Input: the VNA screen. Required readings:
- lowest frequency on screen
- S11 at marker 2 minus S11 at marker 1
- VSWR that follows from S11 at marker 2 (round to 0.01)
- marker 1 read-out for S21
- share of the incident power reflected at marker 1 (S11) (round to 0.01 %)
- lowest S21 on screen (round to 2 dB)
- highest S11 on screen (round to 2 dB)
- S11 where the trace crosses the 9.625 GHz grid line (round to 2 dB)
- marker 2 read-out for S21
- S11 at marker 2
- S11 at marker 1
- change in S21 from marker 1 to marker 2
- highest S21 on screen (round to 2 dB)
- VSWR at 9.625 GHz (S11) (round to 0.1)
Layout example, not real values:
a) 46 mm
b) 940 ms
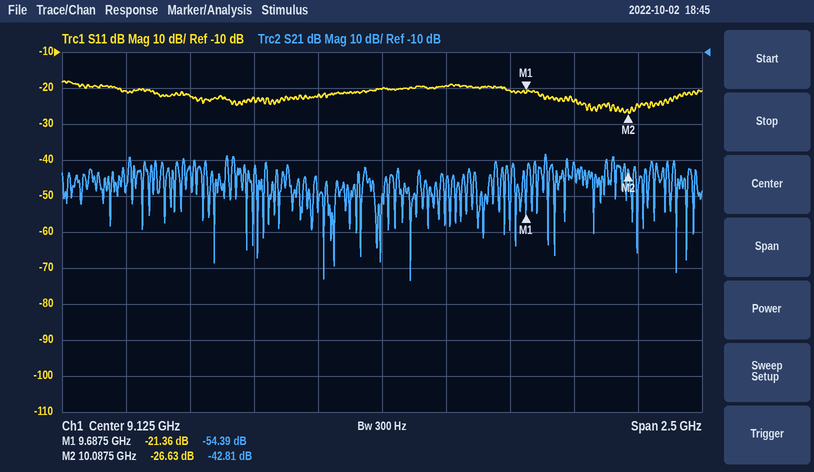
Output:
a) 7.875 GHz
b) -5.27 dB
c) 1.10
d) -54.39 dB
e) 0.73 %
f) -74 dB
g) -18 dB
h) -20 dB
i) -42.81 dB
j) -26.63 dB
k) -21.36 dB
l) 11.58 dB
m) -38 dB
n) 1.2
